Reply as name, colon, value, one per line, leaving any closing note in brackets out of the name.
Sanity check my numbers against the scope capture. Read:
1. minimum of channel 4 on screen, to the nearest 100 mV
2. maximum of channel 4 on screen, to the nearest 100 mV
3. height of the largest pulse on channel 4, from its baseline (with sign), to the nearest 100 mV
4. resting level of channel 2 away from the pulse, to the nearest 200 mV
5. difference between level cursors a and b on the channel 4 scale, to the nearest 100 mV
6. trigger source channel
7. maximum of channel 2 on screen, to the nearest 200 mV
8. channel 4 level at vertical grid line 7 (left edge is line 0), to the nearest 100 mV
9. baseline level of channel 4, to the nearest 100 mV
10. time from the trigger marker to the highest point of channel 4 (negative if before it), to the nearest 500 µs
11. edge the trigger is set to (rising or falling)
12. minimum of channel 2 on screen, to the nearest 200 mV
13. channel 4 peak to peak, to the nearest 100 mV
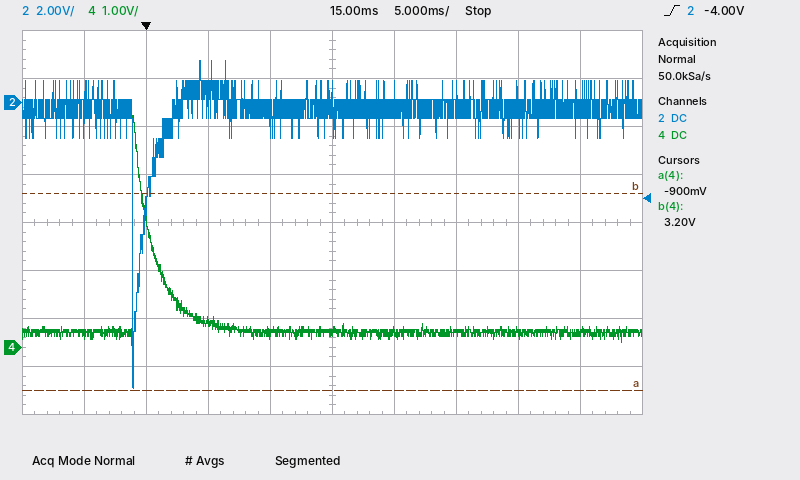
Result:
minimum of channel 4 on screen, to the nearest 100 mV: 0.0 V
maximum of channel 4 on screen, to the nearest 100 mV: 4.8 V
height of the largest pulse on channel 4, from its baseline (with sign), to the nearest 100 mV: +4.5 V
resting level of channel 2 away from the pulse, to the nearest 200 mV: -200 mV
difference between level cursors a and b on the channel 4 scale, to the nearest 100 mV: 4.1 V
trigger source channel: channel 2
maximum of channel 2 on screen, to the nearest 200 mV: 1.8 V
channel 4 level at vertical grid line 7 (left edge is line 0), to the nearest 100 mV: 300 mV
baseline level of channel 4, to the nearest 100 mV: 300 mV
time from the trigger marker to the highest point of channel 4 (negative if before it), to the nearest 500 µs: -1.0 ms
edge the trigger is set to: rising
minimum of channel 2 on screen, to the nearest 200 mV: -12.0 V
channel 4 peak to peak, to the nearest 100 mV: 4.8 V
